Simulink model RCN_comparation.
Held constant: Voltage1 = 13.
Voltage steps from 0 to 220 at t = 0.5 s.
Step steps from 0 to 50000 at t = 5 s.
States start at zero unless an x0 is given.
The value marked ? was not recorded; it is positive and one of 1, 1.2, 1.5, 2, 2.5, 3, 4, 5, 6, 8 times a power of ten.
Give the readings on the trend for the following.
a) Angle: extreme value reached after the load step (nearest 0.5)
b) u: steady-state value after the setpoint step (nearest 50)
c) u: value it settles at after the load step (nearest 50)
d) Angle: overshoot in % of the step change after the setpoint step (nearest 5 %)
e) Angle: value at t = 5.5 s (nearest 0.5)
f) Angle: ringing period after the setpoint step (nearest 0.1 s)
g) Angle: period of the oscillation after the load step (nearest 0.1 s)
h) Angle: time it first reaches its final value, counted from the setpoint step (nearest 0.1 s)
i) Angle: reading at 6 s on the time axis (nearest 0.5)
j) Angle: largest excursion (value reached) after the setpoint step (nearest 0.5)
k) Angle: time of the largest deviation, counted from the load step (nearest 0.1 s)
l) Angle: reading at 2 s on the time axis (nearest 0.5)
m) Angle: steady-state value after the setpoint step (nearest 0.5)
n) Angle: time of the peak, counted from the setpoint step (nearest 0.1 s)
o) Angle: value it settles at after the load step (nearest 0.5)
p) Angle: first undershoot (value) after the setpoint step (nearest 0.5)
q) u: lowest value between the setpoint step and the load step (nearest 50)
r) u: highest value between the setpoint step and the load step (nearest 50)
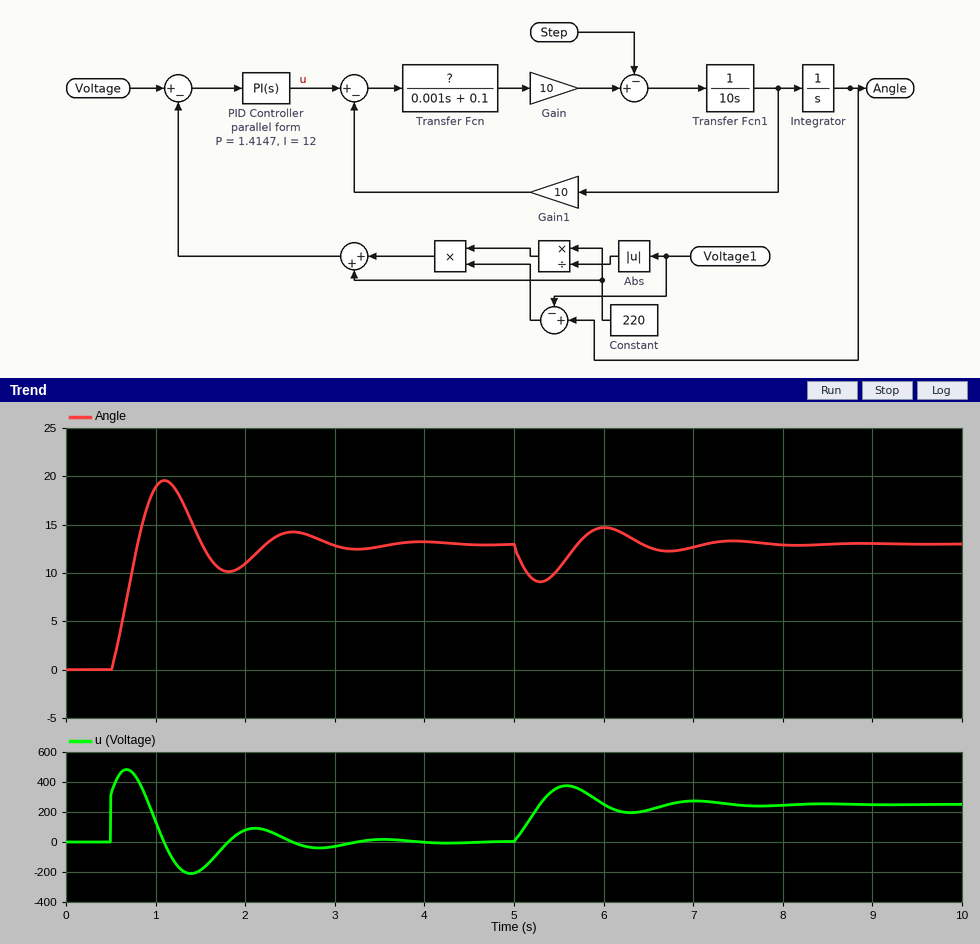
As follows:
9.0
0
250
50 %
10.5
1.4 s
1.4 s
0.3 s
14.5
19.5
0.3 s
11.0
13.0
0.6 s
13.0
10.0
-200
500
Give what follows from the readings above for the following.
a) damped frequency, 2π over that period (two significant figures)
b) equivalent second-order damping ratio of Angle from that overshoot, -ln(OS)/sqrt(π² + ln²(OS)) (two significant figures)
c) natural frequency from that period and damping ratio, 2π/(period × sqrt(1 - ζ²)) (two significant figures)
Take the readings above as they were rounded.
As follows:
4.5 rad/s
0.22
4.6 rad/s
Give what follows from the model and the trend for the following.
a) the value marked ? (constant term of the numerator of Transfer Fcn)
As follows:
2
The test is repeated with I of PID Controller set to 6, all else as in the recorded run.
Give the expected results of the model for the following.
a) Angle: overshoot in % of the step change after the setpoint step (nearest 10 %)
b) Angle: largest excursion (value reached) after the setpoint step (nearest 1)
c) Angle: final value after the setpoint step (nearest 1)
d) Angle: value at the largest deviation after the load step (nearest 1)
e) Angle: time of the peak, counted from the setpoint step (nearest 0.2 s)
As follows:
40 %
18
13
8
0.8 s
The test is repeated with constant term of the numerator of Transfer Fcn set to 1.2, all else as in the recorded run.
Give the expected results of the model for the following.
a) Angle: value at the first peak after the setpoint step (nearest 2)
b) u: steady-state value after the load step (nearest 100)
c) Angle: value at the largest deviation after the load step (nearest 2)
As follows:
20
400
6
